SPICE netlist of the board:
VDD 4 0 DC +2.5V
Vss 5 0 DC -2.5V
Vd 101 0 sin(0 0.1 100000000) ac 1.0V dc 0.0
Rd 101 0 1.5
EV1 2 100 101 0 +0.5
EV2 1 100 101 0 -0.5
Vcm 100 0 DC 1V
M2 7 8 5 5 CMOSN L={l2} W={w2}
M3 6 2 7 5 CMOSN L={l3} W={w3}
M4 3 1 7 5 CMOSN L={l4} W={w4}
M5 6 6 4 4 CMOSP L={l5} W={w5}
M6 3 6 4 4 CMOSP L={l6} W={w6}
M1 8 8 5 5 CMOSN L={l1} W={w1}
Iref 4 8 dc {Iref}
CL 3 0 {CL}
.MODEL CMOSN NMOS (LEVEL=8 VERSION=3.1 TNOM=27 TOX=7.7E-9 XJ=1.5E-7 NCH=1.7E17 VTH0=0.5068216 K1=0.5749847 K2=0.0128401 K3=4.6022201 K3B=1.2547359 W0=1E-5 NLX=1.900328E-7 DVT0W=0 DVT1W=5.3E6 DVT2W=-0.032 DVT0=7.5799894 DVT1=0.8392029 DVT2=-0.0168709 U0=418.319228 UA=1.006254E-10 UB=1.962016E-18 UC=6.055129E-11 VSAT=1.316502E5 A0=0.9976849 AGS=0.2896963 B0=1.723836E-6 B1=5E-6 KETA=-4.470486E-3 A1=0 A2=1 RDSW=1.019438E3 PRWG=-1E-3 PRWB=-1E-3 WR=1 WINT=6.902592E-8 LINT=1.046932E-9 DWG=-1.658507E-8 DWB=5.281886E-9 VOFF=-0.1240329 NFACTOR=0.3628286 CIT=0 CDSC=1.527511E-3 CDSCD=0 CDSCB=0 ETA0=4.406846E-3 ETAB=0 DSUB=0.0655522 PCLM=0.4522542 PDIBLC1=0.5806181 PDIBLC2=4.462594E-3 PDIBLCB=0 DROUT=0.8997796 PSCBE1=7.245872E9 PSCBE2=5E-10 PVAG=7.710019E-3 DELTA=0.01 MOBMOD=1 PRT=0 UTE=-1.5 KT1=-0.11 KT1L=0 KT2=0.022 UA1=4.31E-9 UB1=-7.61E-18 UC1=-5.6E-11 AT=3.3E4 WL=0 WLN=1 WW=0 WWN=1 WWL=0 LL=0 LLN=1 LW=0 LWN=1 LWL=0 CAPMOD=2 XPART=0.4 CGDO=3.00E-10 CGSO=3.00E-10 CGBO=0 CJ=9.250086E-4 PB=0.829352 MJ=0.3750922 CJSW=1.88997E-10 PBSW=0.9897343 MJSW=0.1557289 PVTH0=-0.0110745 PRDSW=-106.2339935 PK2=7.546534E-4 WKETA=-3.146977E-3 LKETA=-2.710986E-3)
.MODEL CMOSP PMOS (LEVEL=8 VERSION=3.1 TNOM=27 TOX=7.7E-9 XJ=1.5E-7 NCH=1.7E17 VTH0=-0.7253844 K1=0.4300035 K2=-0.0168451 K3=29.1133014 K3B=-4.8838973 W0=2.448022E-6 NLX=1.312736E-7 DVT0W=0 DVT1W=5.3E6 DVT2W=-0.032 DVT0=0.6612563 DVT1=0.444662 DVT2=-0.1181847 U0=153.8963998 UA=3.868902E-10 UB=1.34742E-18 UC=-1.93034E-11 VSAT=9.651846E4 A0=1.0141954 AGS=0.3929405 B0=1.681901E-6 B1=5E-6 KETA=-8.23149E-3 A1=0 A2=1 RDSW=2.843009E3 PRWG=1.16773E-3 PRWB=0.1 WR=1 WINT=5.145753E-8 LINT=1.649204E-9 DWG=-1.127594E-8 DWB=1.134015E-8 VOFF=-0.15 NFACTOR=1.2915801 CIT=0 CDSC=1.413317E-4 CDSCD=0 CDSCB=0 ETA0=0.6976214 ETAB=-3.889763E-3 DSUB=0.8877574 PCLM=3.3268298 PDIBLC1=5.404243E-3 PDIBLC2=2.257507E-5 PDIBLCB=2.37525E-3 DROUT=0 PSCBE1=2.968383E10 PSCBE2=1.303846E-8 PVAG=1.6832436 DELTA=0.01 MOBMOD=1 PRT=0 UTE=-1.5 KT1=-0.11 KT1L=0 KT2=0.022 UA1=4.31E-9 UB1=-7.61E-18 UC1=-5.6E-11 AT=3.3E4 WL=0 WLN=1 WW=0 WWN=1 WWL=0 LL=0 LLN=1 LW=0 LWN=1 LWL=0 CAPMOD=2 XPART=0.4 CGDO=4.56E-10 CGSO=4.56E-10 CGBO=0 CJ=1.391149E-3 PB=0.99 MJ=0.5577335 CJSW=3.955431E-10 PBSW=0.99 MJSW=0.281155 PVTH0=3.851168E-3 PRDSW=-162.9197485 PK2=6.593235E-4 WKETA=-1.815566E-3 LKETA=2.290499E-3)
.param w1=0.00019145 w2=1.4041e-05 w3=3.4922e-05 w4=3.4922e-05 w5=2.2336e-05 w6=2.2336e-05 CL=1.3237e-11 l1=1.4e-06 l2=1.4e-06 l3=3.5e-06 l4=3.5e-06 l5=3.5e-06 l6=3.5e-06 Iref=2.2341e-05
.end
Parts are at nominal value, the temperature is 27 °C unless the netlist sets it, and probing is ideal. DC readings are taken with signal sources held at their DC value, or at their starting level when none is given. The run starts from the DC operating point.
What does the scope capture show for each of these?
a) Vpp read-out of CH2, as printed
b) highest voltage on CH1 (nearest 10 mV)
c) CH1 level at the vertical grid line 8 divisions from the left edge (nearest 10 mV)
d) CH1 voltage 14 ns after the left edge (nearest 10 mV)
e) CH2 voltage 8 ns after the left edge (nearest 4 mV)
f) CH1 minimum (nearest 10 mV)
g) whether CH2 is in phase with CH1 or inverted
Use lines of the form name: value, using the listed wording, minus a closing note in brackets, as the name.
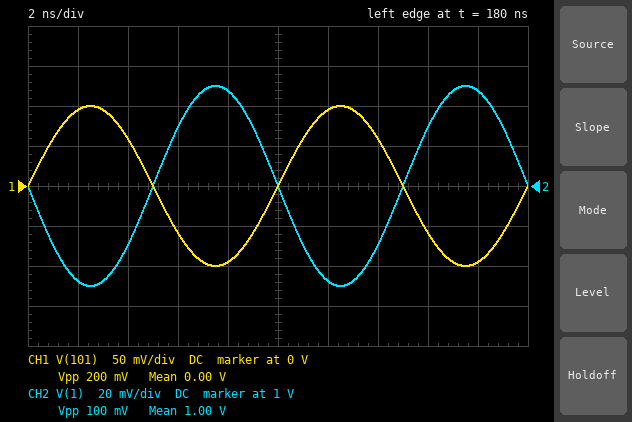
Vpp read-out of CH2, as printed: 100 mV
highest voltage on CH1: 100 mV
CH1 level at the vertical grid line 8 divisions from the left edge: -60 mV
CH1 voltage 14 ns after the left edge: 60 mV
CH2 voltage 8 ns after the left edge: 1.048 V
CH1 minimum: -100 mV
whether CH2 is in phase with CH1 or inverted: inverted
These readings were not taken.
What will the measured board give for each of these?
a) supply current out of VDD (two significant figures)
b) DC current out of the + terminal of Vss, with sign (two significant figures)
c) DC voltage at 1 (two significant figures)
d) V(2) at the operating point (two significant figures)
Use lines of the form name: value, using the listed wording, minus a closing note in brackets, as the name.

supply current out of VDD: 24 µA
DC current out of the + terminal of Vss, with sign: -24 µA
DC voltage at 1: 1.0 V
V(2) at the operating point: 1.0 V
